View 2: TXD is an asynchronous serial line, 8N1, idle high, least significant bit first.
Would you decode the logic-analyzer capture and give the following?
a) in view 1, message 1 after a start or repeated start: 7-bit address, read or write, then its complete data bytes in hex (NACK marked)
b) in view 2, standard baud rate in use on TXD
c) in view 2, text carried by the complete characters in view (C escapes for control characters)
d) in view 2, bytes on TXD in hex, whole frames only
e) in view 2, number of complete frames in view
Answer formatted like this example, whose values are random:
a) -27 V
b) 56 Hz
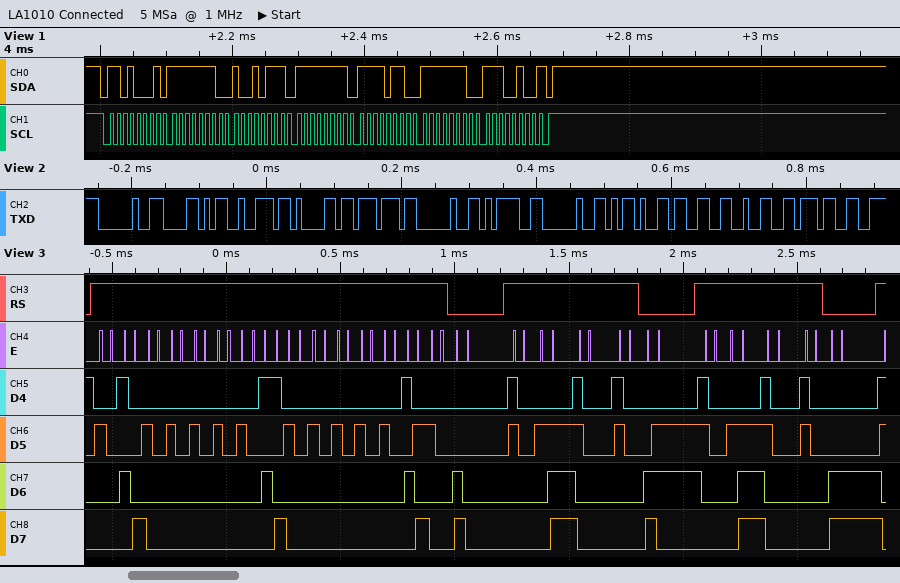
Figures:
a) 0x68 read: FE 97 FF F6 FE E4 NACK
b) 115200 baud
c) " Xraw = -327"
d) 0x20 0x58 0x72 0x61 0x77 0x20 0x3D 0x20 0x2D 0x33 0x32 0x37
e) 12
